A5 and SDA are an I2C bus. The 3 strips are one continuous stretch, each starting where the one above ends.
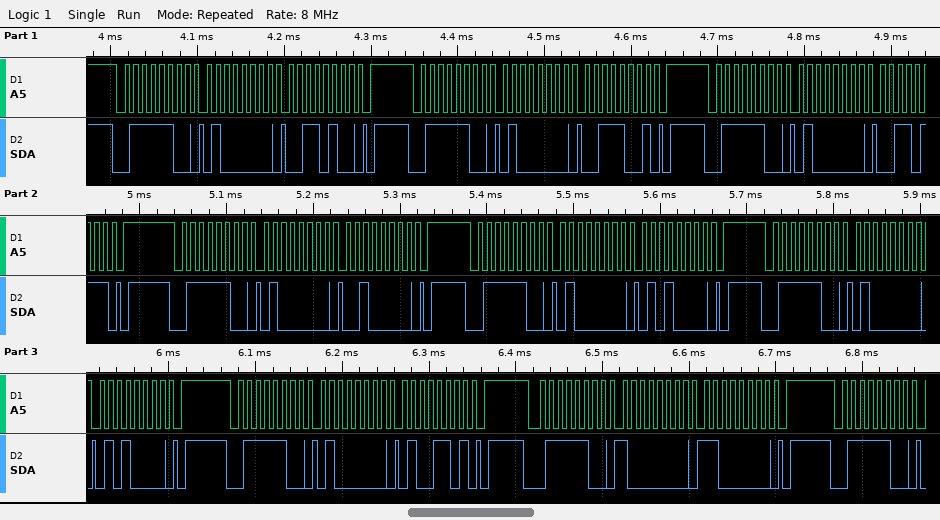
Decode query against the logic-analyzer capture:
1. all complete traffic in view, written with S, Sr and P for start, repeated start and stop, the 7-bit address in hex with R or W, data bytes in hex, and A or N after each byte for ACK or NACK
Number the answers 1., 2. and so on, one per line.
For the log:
1. S 3EW A 40 A 34 A P S 3EW A 40 A 39 A P S 3EW A 40 A 37 A P S 3EW A 40 A 20 A P S 3EW A 40 A 50 A P S 3EW A 40 A 50 A P S 3EW A 40 A 4D A P S 3EW A 80 A C0 A P S 3EW A
